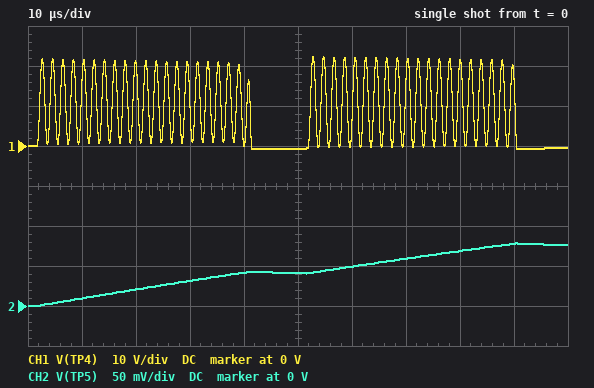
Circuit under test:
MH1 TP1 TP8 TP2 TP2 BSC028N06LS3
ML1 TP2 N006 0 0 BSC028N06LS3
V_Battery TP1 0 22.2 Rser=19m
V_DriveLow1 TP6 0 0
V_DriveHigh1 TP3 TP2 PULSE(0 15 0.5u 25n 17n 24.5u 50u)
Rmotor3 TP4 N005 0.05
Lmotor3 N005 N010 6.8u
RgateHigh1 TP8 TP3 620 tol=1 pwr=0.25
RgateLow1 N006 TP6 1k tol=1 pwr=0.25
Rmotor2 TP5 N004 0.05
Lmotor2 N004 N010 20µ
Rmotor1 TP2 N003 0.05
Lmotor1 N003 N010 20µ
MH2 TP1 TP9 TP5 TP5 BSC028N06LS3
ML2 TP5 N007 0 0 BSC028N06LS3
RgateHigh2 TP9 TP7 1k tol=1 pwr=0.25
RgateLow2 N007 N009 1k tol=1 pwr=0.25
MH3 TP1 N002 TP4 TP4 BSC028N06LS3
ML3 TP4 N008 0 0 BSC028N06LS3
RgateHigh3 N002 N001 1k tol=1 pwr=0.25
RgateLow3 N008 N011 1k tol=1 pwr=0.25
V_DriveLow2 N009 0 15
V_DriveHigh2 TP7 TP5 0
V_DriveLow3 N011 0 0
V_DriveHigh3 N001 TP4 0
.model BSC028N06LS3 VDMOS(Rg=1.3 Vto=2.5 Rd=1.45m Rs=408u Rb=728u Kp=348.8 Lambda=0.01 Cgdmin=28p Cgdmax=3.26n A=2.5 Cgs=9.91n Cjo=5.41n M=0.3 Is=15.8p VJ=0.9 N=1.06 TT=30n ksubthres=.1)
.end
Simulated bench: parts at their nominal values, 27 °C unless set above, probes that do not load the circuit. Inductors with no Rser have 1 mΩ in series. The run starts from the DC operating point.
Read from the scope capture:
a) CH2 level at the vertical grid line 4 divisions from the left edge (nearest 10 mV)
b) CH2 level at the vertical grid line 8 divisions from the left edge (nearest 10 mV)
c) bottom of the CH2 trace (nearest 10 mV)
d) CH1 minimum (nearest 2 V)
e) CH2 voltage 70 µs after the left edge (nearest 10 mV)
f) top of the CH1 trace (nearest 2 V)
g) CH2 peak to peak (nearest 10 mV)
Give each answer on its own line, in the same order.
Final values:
40 mV
70 mV
0 V
0 V
60 mV
22 V
80 mV
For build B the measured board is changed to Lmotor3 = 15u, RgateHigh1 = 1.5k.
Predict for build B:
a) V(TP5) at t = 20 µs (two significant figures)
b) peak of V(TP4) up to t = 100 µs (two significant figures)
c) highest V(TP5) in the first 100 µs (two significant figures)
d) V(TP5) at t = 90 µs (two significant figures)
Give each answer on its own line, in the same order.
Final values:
19 mV
21 V
97 mV
88 mV
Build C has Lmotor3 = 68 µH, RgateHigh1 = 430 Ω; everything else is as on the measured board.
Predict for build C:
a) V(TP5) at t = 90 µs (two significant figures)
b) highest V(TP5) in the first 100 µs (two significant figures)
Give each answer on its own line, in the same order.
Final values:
69 mV
70 mV
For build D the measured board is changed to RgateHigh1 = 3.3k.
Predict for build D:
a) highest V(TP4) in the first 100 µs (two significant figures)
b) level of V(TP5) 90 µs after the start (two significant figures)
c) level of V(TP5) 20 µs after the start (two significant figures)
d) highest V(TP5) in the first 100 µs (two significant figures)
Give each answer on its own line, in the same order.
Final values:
19 V
85 mV
15 mV
94 mV
